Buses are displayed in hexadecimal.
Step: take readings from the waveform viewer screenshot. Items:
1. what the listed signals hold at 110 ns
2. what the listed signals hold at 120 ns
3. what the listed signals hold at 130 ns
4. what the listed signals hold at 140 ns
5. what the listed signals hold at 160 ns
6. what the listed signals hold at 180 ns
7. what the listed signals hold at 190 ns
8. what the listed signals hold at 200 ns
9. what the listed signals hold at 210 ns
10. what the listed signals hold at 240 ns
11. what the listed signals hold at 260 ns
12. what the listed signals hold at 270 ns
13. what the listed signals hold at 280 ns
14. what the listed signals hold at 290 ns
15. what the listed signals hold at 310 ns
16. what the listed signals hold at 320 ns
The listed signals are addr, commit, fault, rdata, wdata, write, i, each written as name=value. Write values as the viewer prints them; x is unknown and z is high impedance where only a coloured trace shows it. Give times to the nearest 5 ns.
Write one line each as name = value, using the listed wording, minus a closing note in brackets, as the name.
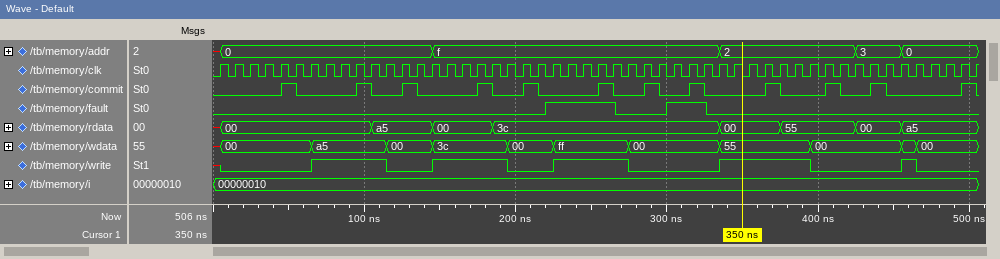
what the listed signals hold at 110 ns = addr=0, commit=0, fault=0, rdata=a5, wdata=a5, write=1, i=00000010
what the listed signals hold at 120 ns = addr=0, commit=0, fault=0, rdata=a5, wdata=00, write=0, i=00000010
what the listed signals hold at 130 ns = addr=0, commit=1, fault=0, rdata=a5, wdata=00, write=0, i=00000010
what the listed signals hold at 140 ns = addr=0, commit=0, fault=0, rdata=a5, wdata=00, write=0, i=00000010
what the listed signals hold at 160 ns = addr=f, commit=0, fault=0, rdata=00, wdata=3c, write=1, i=00000010
what the listed signals hold at 180 ns = addr=f, commit=1, fault=0, rdata=00, wdata=3c, write=1, i=00000010
what the listed signals hold at 190 ns = addr=f, commit=0, fault=0, rdata=3c, wdata=3c, write=1, i=00000010
what the listed signals hold at 200 ns = addr=f, commit=0, fault=0, rdata=3c, wdata=00, write=0, i=00000010
what the listed signals hold at 210 ns = addr=f, commit=1, fault=0, rdata=3c, wdata=00, write=0, i=00000010
what the listed signals hold at 240 ns = addr=f, commit=0, fault=1, rdata=3c, wdata=ff, write=1, i=00000010
what the listed signals hold at 260 ns = addr=f, commit=1, fault=1, rdata=3c, wdata=ff, write=1, i=00000010
what the listed signals hold at 270 ns = addr=f, commit=0, fault=0, rdata=3c, wdata=ff, write=1, i=00000010
what the listed signals hold at 280 ns = addr=f, commit=0, fault=0, rdata=3c, wdata=00, write=0, i=00000010
what the listed signals hold at 290 ns = addr=f, commit=1, fault=0, rdata=3c, wdata=00, write=0, i=00000010
what the listed signals hold at 310 ns = addr=f, commit=0, fault=1, rdata=3c, wdata=00, write=0, i=00000010
what the listed signals hold at 320 ns = addr=f, commit=1, fault=1, rdata=3c, wdata=00, write=0, i=00000010
